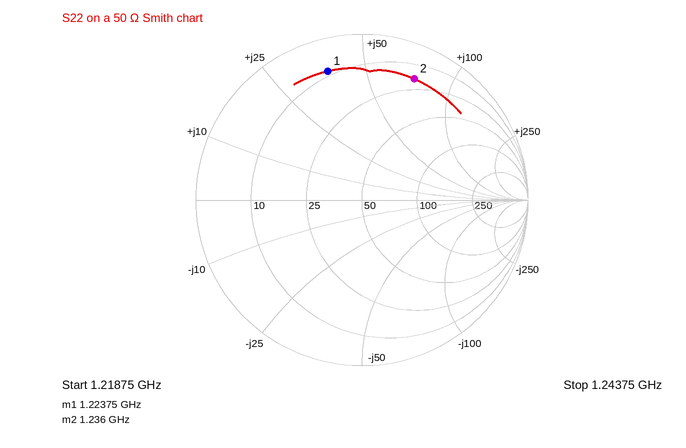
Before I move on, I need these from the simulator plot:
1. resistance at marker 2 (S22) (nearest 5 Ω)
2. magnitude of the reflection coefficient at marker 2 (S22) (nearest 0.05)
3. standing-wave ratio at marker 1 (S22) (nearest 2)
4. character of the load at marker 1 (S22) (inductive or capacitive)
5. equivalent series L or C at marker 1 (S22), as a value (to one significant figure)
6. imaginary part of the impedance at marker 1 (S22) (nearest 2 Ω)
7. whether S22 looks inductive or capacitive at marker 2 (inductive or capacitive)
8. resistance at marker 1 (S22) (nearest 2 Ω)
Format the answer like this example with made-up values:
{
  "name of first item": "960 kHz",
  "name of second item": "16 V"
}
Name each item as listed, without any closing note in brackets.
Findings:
{
  "resistance at marker 2 (S22)": "20 Ω",
  "magnitude of the reflection coefficient at marker 2 (S22)": "0.80",
  "standing-wave ratio at marker 1 (S22)": "10",
  "character of the load at marker 1 (S22)": "inductive",
  "equivalent series L or C at marker 1 (S22), as a value": "5 nH",
  "imaginary part of the impedance at marker 1 (S22)": "+38 Ω",
  "whether S22 looks inductive or capacitive at marker 2": "inductive",
  "resistance at marker 1 (S22)": "8 Ω"
}
